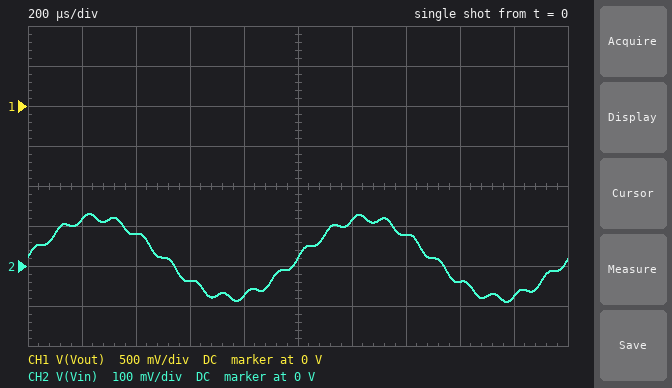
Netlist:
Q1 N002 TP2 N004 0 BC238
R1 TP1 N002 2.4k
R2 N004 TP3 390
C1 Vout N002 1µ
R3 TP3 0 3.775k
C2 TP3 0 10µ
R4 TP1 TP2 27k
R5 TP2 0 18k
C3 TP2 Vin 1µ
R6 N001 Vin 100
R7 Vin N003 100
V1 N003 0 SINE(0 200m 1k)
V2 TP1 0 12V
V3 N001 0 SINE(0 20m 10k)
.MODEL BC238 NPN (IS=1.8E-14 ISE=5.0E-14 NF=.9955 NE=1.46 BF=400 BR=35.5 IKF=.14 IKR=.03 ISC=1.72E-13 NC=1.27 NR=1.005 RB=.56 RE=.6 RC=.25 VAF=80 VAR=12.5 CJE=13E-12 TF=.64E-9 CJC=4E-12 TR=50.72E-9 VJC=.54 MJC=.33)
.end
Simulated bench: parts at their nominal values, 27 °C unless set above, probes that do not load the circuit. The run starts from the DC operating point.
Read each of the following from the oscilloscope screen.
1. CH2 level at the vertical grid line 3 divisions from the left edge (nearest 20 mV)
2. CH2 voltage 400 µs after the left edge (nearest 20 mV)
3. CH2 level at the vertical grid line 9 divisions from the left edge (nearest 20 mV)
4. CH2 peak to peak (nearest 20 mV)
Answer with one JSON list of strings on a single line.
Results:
["-40 mV", "80 mV", "-80 mV", "220 mV"]
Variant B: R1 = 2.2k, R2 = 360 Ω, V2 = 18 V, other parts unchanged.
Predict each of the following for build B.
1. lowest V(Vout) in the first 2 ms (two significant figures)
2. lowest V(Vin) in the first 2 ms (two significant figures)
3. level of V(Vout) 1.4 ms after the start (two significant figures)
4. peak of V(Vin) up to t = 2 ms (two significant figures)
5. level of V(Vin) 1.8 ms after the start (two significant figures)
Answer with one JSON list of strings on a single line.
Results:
["15 V", "-80 mV", "16 V", "140 mV", "-67 mV"]
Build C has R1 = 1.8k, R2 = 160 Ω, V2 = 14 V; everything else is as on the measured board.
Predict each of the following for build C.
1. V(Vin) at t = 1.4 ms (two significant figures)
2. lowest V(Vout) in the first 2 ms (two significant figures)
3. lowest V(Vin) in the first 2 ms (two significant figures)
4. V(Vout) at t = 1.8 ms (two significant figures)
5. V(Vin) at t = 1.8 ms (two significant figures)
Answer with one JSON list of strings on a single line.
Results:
["81 mV", "11 V", "-87 mV", "13 V", "-73 mV"]
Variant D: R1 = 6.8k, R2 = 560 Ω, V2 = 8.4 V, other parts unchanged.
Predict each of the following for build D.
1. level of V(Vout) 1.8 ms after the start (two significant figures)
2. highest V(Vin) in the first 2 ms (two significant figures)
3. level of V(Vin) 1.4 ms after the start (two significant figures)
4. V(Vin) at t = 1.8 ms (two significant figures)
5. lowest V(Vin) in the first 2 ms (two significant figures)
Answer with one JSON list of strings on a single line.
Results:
["8.4 V", "120 mV", "72 mV", "-82 mV", "-95 mV"]
